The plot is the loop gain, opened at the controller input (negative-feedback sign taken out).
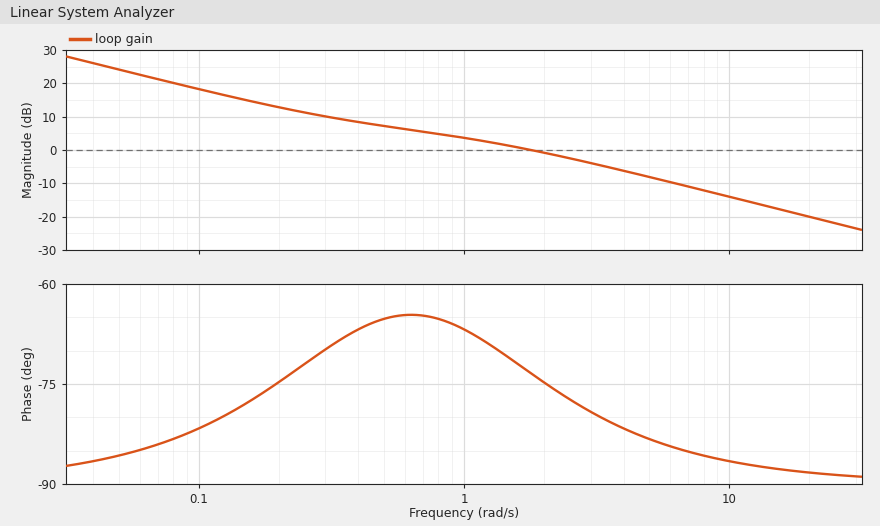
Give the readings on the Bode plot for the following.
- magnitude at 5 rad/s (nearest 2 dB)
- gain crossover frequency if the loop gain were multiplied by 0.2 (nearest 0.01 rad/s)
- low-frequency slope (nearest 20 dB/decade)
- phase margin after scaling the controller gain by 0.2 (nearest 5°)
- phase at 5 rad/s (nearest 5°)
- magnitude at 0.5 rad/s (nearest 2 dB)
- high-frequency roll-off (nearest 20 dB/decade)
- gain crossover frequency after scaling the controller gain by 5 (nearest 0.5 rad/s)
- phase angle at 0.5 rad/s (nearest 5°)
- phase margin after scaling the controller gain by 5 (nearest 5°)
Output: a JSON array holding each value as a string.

["-8 dB", "0.17 rad/s", "-20 dB/decade", "105°", "-85°", "8 dB", "-20 dB/decade", "10.0 rad/s", "-65°", "95°"]
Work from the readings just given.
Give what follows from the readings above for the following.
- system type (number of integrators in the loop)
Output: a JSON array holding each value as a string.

["1"]
